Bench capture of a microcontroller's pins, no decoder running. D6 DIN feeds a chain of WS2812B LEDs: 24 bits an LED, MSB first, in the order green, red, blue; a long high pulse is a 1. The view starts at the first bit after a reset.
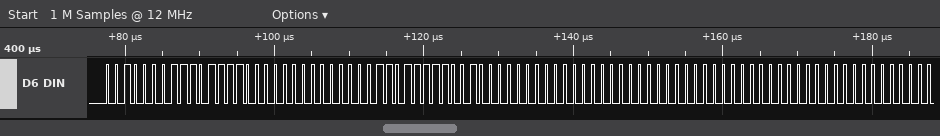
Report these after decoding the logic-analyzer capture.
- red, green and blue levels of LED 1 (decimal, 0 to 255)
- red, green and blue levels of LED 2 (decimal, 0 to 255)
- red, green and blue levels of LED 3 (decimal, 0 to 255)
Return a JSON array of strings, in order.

["222, 33, 0", "249, 6, 0", "0, 0, 0"]
